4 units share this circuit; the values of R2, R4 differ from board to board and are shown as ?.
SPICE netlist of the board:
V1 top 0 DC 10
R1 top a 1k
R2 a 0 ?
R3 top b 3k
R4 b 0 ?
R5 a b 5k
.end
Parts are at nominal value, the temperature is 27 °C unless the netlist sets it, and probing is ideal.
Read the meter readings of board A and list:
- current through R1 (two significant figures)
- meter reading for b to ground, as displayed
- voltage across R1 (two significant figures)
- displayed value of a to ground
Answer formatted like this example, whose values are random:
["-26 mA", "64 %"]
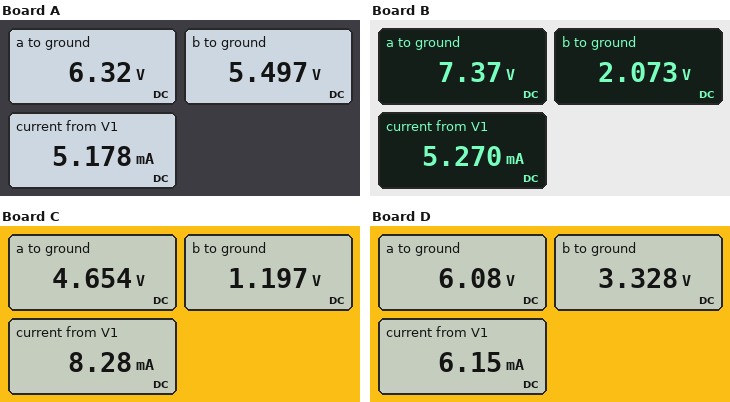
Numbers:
["3.7 mA", "5.497 V", "3.7 V", "6.32 V"]
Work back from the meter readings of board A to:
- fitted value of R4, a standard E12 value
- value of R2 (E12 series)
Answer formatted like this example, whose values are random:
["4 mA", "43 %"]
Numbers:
["3.3 kΩ", "1.8 kΩ"]
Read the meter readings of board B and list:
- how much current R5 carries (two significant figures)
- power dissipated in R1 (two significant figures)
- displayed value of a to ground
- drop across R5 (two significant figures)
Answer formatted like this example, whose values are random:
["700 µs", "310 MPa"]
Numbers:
["1.1 mA", "6.9 mW", "7.37 V", "5.3 V"]
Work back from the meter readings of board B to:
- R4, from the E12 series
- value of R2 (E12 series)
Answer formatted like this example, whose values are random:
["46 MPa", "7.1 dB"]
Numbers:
["560 Ω", "4.7 kΩ"]
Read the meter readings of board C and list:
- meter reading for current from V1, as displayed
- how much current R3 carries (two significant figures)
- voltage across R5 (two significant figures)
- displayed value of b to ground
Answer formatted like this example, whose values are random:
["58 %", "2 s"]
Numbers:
["8.28 mA", "2.9 mA", "3.5 V", "1.197 V"]
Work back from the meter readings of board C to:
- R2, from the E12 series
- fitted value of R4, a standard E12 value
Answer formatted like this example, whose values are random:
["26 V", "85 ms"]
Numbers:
["1 kΩ", "330 Ω"]
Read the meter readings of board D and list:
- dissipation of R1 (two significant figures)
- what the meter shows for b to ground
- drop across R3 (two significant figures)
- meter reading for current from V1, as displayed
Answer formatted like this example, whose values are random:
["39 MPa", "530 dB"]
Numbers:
["15 mW", "3.328 V", "6.7 V", "6.15 mA"]
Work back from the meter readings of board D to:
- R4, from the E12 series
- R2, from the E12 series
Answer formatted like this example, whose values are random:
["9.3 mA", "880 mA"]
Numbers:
["1.2 kΩ", "1.8 kΩ"]
